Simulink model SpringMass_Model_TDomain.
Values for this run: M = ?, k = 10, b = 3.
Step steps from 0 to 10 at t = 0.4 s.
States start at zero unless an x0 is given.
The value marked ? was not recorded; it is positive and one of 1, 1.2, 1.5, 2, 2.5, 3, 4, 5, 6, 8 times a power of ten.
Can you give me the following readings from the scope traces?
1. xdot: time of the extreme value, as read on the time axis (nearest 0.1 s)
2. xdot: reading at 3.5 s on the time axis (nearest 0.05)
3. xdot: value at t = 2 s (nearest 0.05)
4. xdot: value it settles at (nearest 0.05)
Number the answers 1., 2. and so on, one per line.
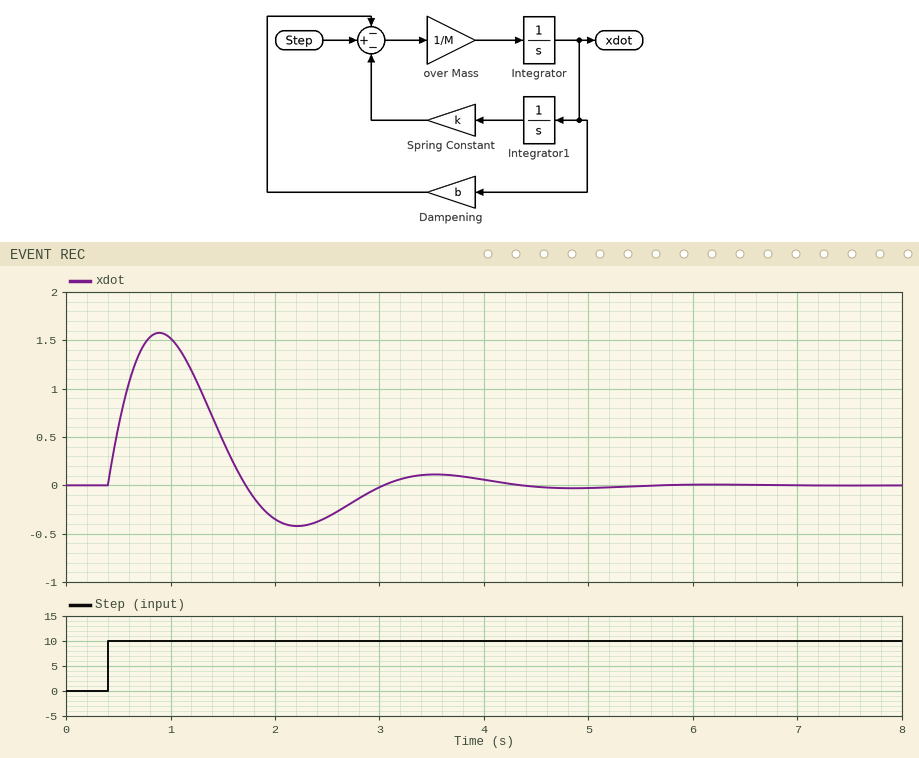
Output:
1. 0.9 s
2. 0.10
3. -0.35
4. 0.00
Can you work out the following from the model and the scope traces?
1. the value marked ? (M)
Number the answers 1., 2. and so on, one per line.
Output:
1. 1.5
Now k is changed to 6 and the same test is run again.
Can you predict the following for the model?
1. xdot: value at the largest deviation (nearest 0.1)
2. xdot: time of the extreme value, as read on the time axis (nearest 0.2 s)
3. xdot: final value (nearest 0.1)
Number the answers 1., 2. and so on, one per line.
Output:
1. 1.8
2. 1.0 s
3. 0.0
